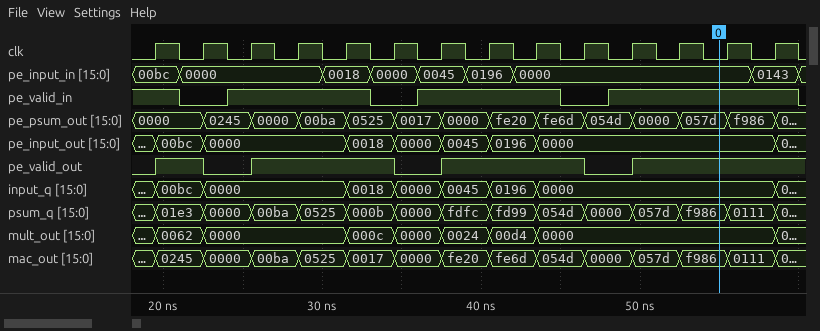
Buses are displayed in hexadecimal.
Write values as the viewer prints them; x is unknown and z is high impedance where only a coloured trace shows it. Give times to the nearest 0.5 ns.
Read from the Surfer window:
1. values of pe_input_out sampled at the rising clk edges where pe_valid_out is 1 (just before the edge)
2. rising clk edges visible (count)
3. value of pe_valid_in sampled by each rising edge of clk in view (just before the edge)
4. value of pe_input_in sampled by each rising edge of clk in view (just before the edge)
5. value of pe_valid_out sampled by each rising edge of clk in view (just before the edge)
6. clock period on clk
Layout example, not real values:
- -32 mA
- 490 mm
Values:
- 00bc, 0000, 0000, 0018, 0045, 0196, 0000, 0000, 0000, 0000
- 14
- 1 0 1 1 1 0 1 1 1 0 1 1 1 1
- 00bc, 0000, 0000, 0000, 0018, 0000, 0045, 0196, 0000, 0000, 0000, 0000, 0000, 0143
- 0 1 0 1 1 1 0 1 1 1 0 1 1 1
- 3 ns
